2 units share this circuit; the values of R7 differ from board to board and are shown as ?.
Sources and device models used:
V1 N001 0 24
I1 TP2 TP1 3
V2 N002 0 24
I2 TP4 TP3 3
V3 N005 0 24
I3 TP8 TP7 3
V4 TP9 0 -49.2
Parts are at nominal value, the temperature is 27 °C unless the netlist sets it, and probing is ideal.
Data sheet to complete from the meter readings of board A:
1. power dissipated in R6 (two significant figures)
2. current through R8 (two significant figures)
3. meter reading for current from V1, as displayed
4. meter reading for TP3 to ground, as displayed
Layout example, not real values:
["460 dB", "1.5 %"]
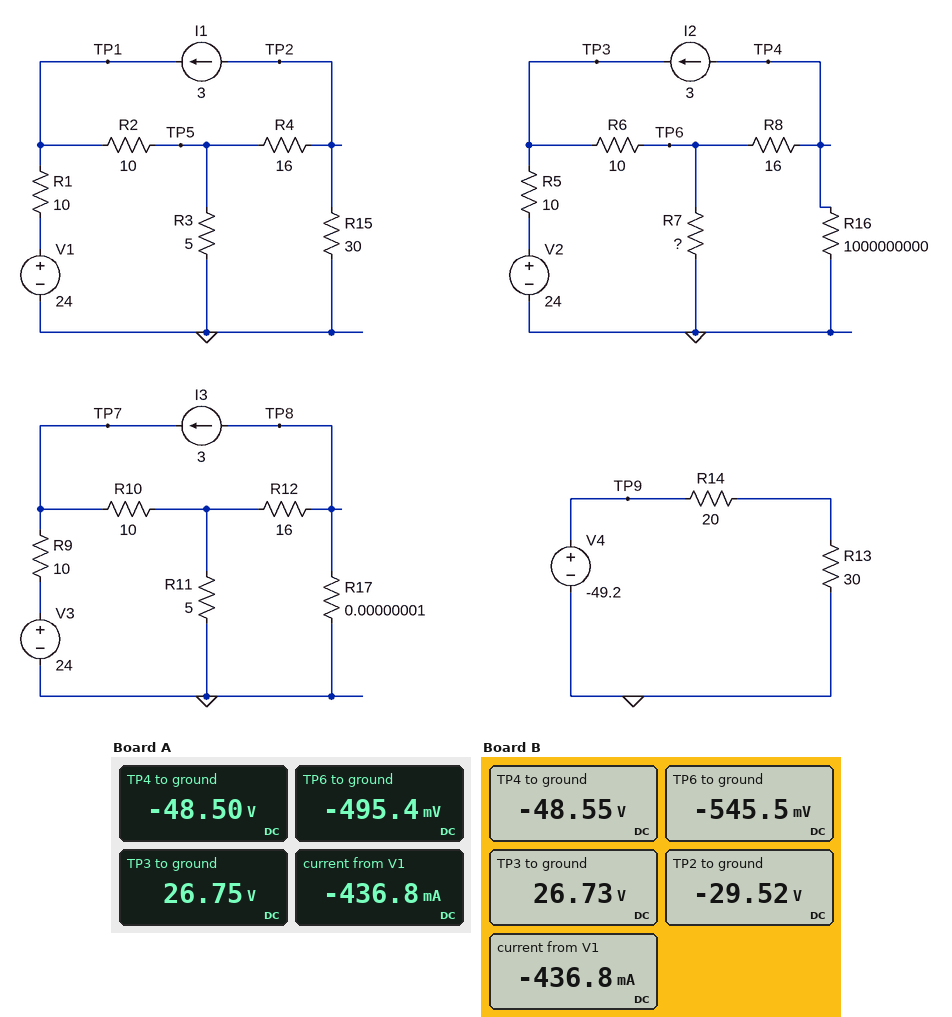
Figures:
["74 W", "3.0 A", "-436.8 mA", "26.75 V"]
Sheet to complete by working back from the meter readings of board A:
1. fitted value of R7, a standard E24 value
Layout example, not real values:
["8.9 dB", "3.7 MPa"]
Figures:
["1.8 Ω"]
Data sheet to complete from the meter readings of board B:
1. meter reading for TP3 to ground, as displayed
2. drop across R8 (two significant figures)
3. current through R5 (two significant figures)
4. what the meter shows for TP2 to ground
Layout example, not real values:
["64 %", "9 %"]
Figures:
["26.73 V", "48 V", "270 mA", "-29.52 V"]
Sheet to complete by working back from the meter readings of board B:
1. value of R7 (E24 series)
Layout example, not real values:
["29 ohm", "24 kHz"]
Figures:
["2 Ω"]
